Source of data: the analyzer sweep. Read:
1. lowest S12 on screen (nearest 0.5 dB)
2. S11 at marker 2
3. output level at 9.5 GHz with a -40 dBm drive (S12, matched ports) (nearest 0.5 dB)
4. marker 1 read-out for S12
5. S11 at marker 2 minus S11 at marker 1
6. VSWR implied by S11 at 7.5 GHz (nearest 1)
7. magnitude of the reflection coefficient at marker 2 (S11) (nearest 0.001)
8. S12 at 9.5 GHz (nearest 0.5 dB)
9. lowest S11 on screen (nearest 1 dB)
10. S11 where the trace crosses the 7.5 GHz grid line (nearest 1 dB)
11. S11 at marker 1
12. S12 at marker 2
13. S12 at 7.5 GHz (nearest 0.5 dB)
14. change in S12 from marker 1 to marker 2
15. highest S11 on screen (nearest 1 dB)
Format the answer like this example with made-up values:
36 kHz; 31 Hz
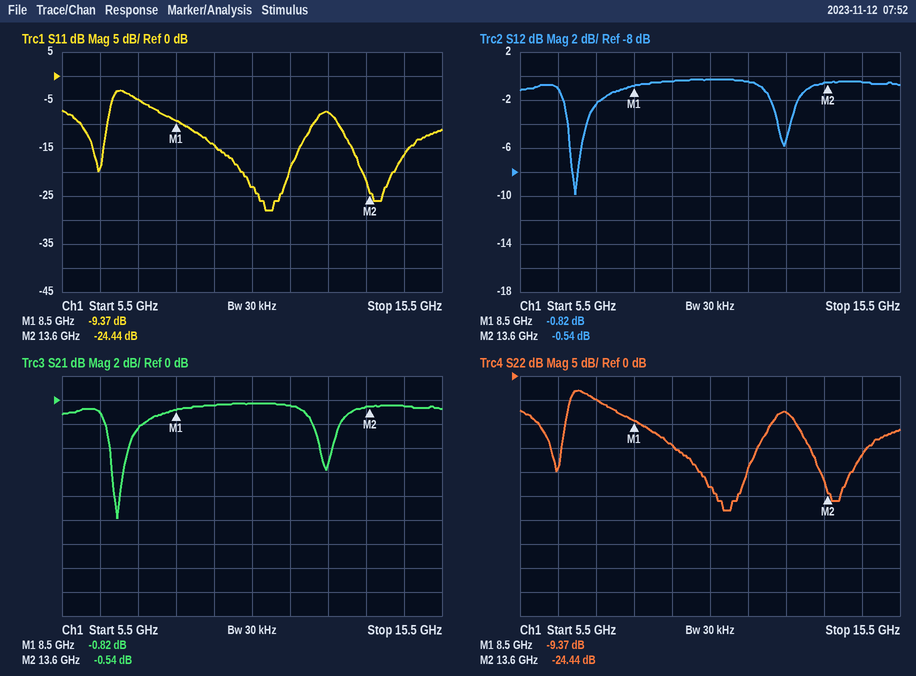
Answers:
-10.0 dB; -24.44 dB; -40.5 dBm; -0.82 dB; -15.07 dB; 4; 0.060; -0.5 dB; -28 dB; -5 dB; -9.37 dB; -0.54 dB; -2.5 dB; 0.28 dB; -3 dB
